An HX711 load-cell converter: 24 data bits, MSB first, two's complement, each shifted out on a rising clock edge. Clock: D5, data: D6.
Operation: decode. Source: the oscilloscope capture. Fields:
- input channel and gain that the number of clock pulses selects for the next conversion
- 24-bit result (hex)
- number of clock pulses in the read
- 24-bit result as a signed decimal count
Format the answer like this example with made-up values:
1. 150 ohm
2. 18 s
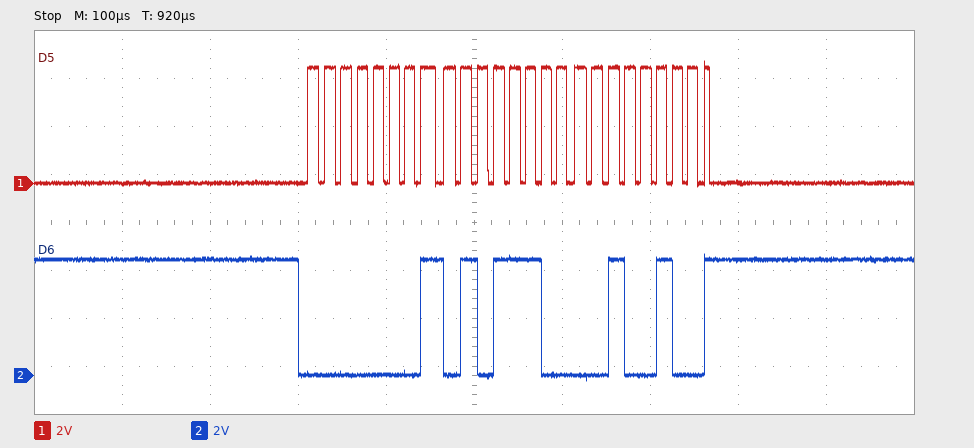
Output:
1. channel A, gain 128
2. 0x015C24
3. 25
4. 89124
